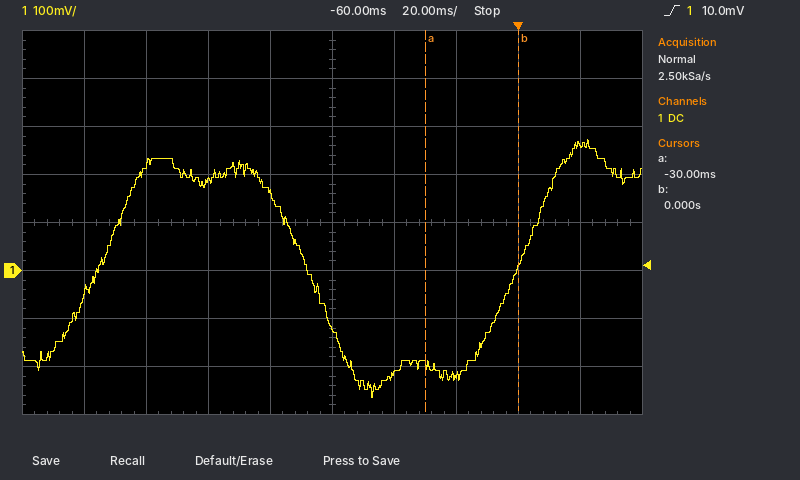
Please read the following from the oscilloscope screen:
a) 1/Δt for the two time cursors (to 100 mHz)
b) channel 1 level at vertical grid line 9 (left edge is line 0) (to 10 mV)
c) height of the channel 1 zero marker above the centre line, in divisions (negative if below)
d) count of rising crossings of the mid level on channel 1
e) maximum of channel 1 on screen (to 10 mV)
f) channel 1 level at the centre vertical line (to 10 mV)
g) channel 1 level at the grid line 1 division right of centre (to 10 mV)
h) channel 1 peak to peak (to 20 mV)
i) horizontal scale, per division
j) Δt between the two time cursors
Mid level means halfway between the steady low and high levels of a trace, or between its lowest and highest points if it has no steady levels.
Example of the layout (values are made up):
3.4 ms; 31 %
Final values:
33.3 Hz; 260 mV; -1.0 div; 2; 270 mV; -120 mV; -220 mV; 540 mV; 20 ms; 30 ms
